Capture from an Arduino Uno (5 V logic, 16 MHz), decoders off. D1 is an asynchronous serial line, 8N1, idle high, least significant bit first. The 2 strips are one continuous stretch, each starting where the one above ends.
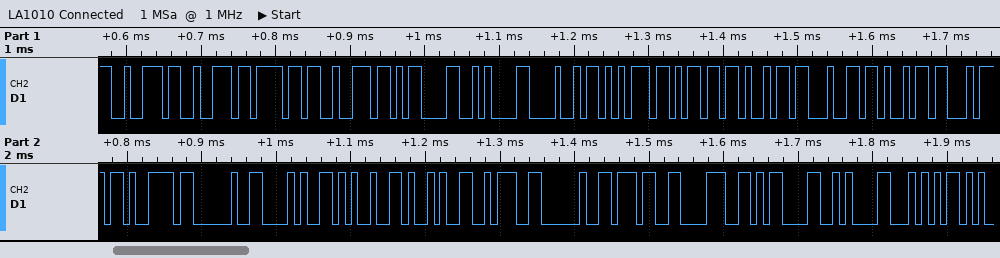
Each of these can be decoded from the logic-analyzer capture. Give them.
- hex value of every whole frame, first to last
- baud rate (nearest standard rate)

72 72 6F 72 0D 0A 48 75 6D 69 64 69 74 79 20 28 25 29 3A 20 37 38 0D 0A 54
115200 baud
